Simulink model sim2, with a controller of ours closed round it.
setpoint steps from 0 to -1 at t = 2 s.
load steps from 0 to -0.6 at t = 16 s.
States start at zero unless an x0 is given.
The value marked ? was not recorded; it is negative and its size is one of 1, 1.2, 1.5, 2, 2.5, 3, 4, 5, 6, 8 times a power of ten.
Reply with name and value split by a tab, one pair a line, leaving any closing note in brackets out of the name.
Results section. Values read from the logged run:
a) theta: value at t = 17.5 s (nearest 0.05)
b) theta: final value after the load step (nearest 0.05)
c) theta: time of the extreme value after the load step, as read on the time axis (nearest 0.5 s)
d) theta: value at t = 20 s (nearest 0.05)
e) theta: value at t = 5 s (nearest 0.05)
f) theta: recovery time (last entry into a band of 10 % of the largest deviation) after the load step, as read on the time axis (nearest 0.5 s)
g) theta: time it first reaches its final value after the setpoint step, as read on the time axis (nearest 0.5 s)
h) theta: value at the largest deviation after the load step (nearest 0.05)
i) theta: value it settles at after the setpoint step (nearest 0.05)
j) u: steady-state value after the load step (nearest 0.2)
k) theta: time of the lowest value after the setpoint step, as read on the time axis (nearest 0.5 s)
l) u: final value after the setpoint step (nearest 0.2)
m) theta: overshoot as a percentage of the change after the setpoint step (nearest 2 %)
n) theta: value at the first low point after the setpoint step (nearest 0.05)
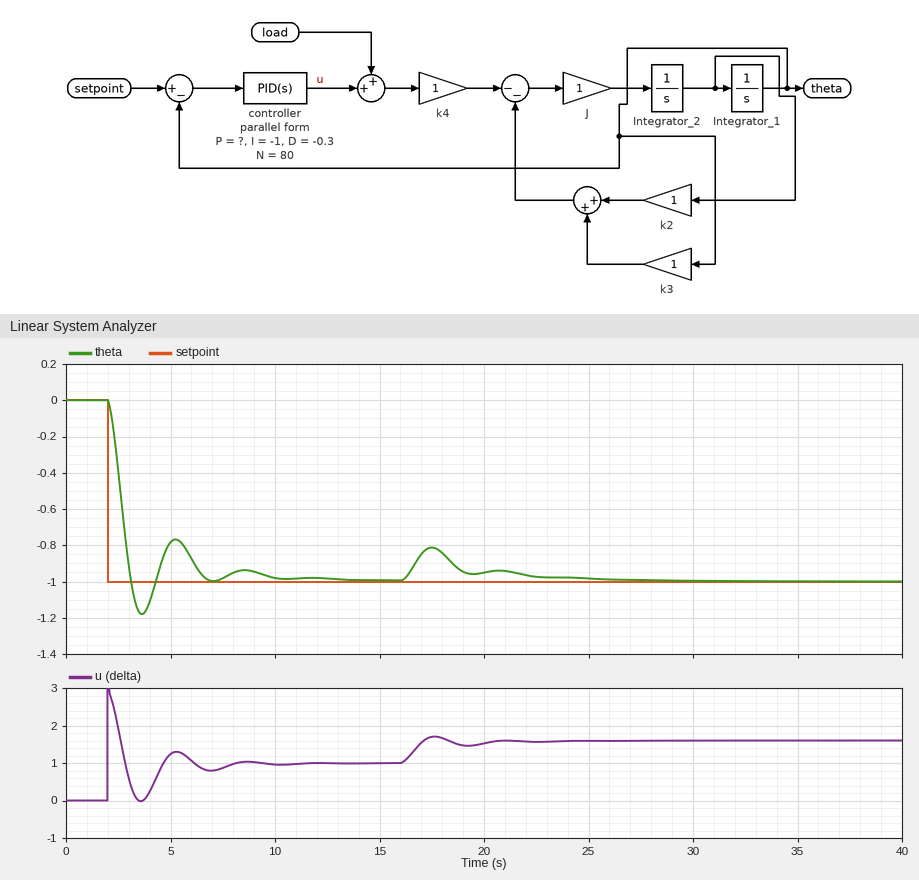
theta: value at t = 17.5 s	-0.80
theta: final value after the load step	-1.00
theta: time of the extreme value after the load step, as read on the time axis	17.5 s
theta: value at t = 20 s	-0.95
theta: value at t = 5 s	-0.80
theta: recovery time (last entry into a band of 10 % of the largest deviation) after the load step, as read on the time axis	25.0 s
theta: time it first reaches its final value after the setpoint step, as read on the time axis	3.0 s
theta: value at the largest deviation after the load step	-0.80
theta: value it settles at after the setpoint step	-1.00
u: steady-state value after the load step	1.6
theta: time of the lowest value after the setpoint step, as read on the time axis	3.5 s
u: final value after the setpoint step	1.0
theta: overshoot as a percentage of the change after the setpoint step	18 %
theta: value at the first low point after the setpoint step	-1.20
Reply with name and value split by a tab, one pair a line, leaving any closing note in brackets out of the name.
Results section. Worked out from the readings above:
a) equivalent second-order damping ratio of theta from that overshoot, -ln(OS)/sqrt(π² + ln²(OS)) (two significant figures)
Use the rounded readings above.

equivalent second-order damping ratio of theta from that overshoot, -ln(OS)/sqrt(π² + ln²(OS))	0.48
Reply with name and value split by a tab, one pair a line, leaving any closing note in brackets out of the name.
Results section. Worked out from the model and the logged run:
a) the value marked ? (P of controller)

the value marked ?	-3
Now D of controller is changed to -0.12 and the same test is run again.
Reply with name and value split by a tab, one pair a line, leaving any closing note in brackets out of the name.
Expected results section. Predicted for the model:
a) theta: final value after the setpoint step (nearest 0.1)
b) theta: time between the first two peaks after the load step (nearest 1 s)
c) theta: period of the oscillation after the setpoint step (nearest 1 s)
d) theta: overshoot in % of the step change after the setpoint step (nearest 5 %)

theta: final value after the setpoint step	-1.0
theta: time between the first two peaks after the load step	3 s
theta: period of the oscillation after the setpoint step	3 s
theta: overshoot in % of the step change after the setpoint step	25 %
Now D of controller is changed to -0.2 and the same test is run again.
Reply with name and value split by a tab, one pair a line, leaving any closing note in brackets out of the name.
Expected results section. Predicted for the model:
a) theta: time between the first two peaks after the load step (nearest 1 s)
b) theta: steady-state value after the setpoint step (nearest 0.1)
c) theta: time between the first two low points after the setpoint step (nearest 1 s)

theta: time between the first two peaks after the load step	3 s
theta: steady-state value after the setpoint step	-1.0
theta: time between the first two low points after the setpoint step	3 s
